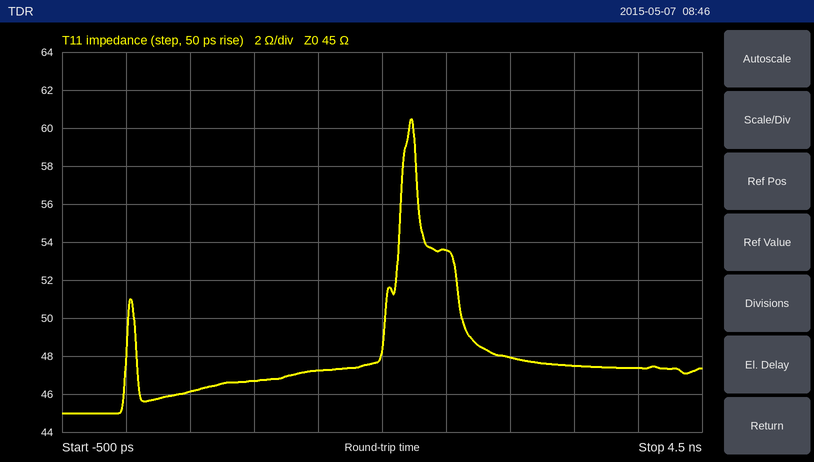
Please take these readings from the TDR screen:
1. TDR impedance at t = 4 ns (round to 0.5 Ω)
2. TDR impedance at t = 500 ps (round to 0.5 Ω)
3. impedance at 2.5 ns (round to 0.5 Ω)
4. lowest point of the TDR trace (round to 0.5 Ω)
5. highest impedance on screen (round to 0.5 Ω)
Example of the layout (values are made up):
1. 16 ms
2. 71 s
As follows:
1. 47.5 Ω
2. 46.0 Ω
3. 53.5 Ω
4. 45.0 Ω
5. 60.5 Ω
